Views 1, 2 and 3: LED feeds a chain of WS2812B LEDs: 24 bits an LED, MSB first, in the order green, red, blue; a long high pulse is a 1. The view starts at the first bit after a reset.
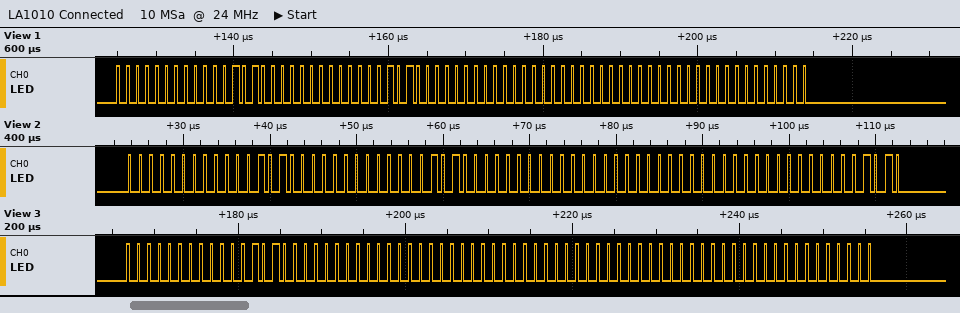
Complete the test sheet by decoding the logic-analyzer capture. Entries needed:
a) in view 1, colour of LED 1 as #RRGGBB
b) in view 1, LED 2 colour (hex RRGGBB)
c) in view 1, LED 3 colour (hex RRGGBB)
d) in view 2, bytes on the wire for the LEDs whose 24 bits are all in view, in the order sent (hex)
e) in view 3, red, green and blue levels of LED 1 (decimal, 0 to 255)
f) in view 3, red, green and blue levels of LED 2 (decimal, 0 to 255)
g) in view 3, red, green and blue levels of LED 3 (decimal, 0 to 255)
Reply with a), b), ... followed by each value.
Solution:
a) #0A0000
b) #000A00
c) #000000
d) 00 0A 00 0A 00 00 00 00 0A
e) 10, 0, 0
f) 0, 0, 0
g) 0, 0, 0
